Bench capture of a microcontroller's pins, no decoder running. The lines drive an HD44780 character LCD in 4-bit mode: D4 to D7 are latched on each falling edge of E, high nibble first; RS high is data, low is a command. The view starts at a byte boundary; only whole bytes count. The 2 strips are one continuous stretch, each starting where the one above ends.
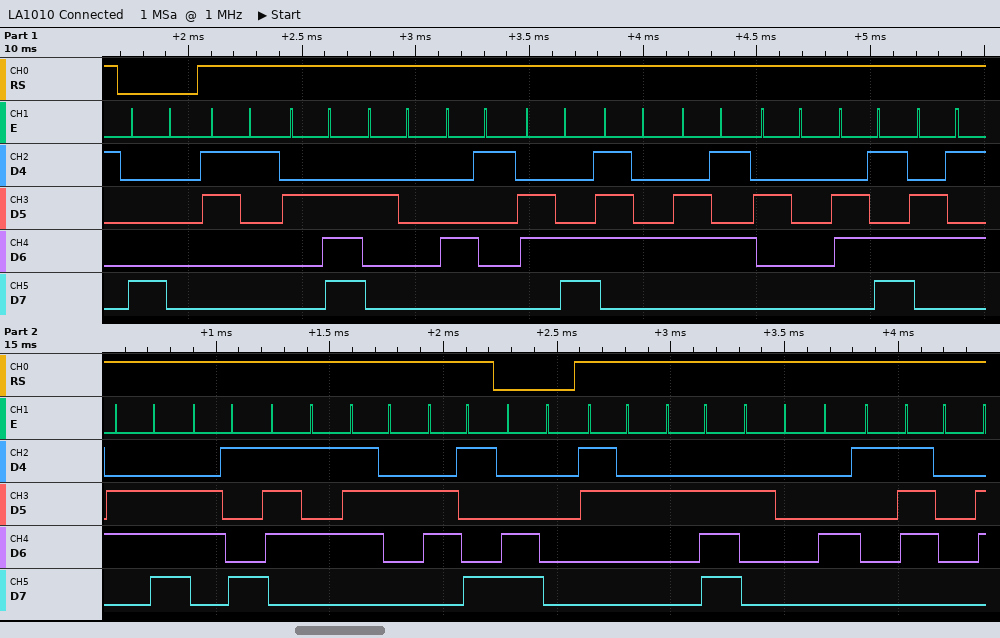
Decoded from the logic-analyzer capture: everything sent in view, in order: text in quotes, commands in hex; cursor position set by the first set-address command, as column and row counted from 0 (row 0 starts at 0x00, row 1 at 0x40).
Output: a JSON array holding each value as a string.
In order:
["0x80 \"1. Alte meniuri\" 0xC0 \"2. Ap\"", "column 0, row 0"]
